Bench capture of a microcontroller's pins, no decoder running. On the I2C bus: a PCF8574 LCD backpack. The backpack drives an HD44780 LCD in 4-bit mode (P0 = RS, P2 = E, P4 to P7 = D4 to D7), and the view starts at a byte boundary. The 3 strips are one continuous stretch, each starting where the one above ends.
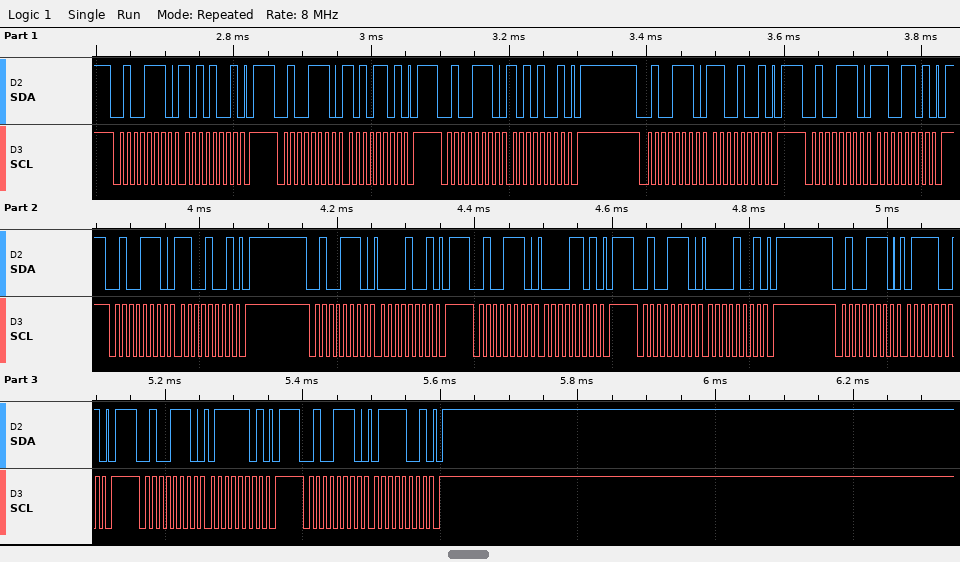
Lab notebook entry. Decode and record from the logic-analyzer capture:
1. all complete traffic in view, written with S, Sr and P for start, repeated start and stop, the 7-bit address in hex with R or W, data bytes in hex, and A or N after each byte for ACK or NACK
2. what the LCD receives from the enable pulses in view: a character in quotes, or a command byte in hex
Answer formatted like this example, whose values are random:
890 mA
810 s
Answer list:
S 27W A A9 A P S 27W A AD A P S 27W A A9 A P S 27W A C9 A P S 27W A CD A P S 27W A C9 A P S 27W A 09 A P S 27W A 0D A P S 27W A 09 A P S 27W A 79 A P S 27W A 7D A P S 27W A 79 A P
data 0xAC data 0x07
